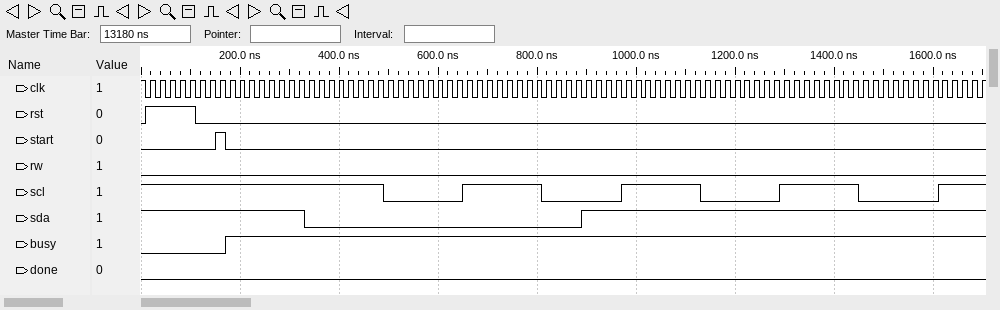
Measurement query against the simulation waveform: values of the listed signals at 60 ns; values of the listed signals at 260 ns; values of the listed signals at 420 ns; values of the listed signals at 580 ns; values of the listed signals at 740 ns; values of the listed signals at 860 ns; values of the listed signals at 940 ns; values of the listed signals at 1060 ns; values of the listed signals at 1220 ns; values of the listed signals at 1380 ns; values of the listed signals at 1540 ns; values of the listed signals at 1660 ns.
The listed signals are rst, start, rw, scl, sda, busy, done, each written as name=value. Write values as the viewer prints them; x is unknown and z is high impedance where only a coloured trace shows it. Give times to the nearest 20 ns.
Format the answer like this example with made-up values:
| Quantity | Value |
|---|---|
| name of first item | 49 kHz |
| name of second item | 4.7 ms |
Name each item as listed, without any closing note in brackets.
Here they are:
| Quantity | Value |
|---|---|
| values of the listed signals at 60 ns | rst=1, start=0, rw=0, scl=1, sda=1, busy=0, done=0 |
| values of the listed signals at 260 ns | rst=0, start=0, rw=0, scl=1, sda=1, busy=1, done=0 |
| values of the listed signals at 420 ns | rst=0, start=0, rw=0, scl=1, sda=0, busy=1, done=0 |
| values of the listed signals at 580 ns | rst=0, start=0, rw=0, scl=0, sda=0, busy=1, done=0 |
| values of the listed signals at 740 ns | rst=0, start=0, rw=0, scl=1, sda=0, busy=1, done=0 |
| values of the listed signals at 860 ns | rst=0, start=0, rw=0, scl=0, sda=0, busy=1, done=0 |
| values of the listed signals at 940 ns | rst=0, start=0, rw=0, scl=0, sda=1, busy=1, done=0 |
| values of the listed signals at 1060 ns | rst=0, start=0, rw=0, scl=1, sda=1, busy=1, done=0 |
| values of the listed signals at 1220 ns | rst=0, start=0, rw=0, scl=0, sda=1, busy=1, done=0 |
| values of the listed signals at 1380 ns | rst=0, start=0, rw=0, scl=1, sda=1, busy=1, done=0 |
| values of the listed signals at 1540 ns | rst=0, start=0, rw=0, scl=0, sda=1, busy=1, done=0 |
| values of the listed signals at 1660 ns | rst=0, start=0, rw=0, scl=1, sda=1, busy=1, done=0 |
